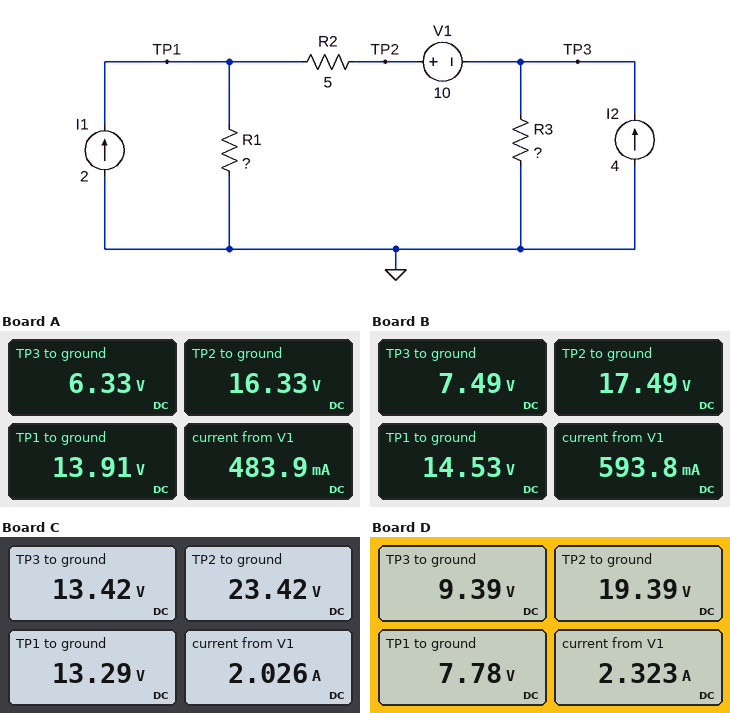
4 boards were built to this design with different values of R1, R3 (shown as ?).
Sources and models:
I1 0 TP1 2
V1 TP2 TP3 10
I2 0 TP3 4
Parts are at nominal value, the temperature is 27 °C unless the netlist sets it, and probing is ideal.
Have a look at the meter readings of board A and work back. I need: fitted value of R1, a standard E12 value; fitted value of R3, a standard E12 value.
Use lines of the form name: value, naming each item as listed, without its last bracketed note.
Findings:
fitted value of R1, a standard E12 value: 5.6 Ω
fitted value of R3, a standard E12 value: 1.8 Ω
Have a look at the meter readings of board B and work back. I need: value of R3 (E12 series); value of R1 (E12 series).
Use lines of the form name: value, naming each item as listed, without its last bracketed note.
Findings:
value of R3: 2.2 Ω
value of R1: 5.6 Ω
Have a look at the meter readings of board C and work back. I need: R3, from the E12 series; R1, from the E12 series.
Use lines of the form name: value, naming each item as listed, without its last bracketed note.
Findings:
R3, from the E12 series: 6.8 Ω
R1, from the E12 series: 3.3 Ω
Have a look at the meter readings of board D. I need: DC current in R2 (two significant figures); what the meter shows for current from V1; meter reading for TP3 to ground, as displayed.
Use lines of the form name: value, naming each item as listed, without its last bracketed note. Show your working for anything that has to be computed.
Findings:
DC current in R2: (19.39 V - 7.78 V) / 5 Ω = 2.3 A
what the meter shows for current from V1: 2.323 A
meter reading for TP3 to ground, as displayed: 9.39 V
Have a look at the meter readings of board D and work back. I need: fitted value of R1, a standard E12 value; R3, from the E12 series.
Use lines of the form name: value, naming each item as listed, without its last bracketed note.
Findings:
fitted value of R1, a standard E12 value: 1.8 Ω
R3, from the E12 series: 5.6 Ω
